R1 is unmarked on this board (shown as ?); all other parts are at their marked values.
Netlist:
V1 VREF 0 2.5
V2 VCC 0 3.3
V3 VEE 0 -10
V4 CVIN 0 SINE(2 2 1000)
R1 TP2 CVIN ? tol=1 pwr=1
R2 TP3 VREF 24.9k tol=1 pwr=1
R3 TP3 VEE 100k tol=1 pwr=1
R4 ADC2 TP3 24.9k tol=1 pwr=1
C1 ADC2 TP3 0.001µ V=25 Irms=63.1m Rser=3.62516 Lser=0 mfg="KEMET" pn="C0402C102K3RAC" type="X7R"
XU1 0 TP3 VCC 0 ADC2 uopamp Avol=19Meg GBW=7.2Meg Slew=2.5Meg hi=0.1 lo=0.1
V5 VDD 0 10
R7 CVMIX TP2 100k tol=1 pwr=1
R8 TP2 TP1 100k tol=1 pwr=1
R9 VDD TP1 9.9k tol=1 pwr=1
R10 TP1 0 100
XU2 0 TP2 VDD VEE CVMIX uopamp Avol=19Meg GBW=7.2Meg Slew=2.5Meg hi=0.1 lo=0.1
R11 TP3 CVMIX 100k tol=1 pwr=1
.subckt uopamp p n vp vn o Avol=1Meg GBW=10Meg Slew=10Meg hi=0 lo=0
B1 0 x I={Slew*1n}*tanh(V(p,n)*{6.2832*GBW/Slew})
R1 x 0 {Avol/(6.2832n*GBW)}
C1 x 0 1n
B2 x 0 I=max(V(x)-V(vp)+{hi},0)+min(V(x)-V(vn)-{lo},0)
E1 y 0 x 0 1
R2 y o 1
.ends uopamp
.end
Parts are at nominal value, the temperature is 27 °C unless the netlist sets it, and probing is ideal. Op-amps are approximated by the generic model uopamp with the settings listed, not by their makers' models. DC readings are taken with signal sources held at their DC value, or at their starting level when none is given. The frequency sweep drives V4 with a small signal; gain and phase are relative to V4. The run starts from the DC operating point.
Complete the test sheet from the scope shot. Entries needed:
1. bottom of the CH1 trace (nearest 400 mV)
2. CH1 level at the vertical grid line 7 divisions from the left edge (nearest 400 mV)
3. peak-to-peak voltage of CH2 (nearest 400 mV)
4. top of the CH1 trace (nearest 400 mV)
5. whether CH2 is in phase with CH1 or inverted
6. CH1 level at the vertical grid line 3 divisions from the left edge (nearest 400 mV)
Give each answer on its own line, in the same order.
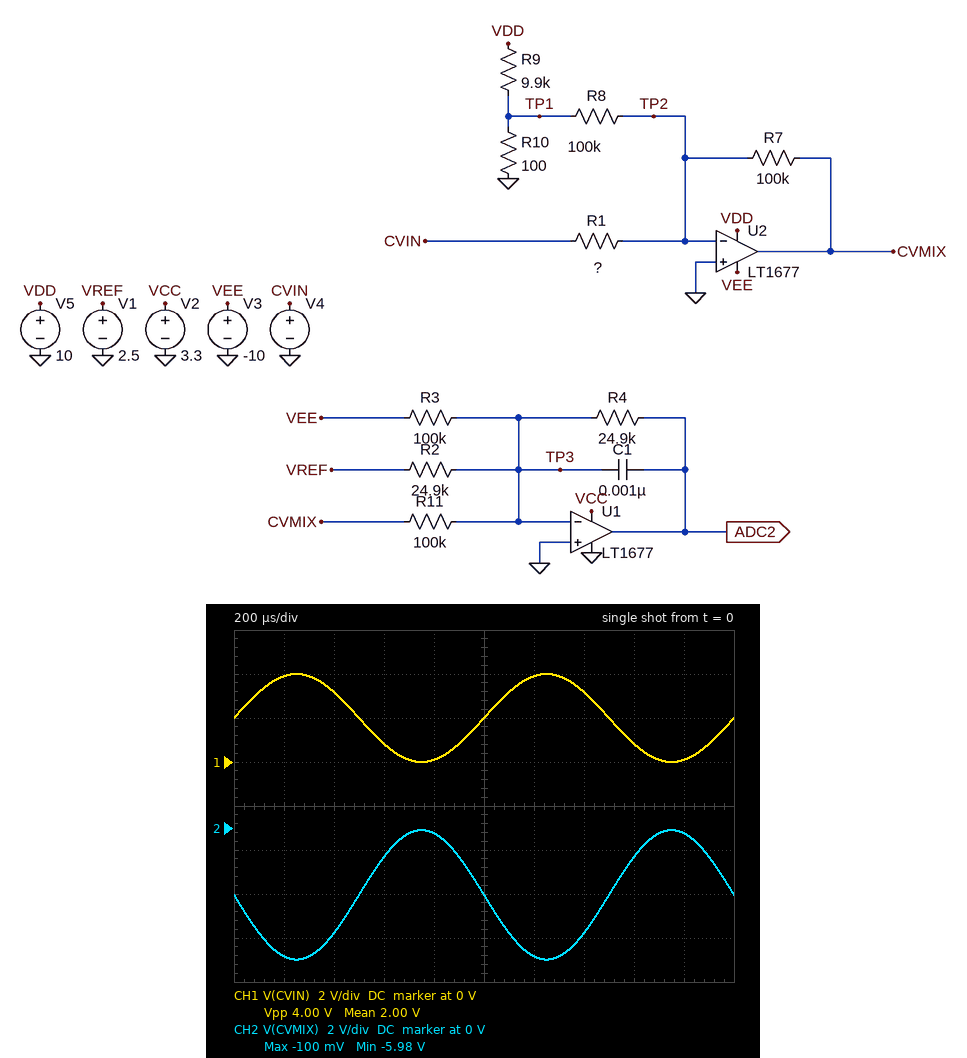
0 V
3.2 V
6.0 V
4.0 V
inverted
800 mV
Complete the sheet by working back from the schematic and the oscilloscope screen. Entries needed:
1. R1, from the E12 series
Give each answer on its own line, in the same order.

68 kΩ
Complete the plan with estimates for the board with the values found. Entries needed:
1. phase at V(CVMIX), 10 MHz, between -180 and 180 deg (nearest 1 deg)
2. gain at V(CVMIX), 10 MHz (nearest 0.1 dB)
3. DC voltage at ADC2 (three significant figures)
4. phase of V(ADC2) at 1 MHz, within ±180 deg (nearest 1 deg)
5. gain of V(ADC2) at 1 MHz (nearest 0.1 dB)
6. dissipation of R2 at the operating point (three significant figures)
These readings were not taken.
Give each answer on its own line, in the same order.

102 deg
-10.5 dB
747 mV
-122 deg
-53.6 dB
251 µW
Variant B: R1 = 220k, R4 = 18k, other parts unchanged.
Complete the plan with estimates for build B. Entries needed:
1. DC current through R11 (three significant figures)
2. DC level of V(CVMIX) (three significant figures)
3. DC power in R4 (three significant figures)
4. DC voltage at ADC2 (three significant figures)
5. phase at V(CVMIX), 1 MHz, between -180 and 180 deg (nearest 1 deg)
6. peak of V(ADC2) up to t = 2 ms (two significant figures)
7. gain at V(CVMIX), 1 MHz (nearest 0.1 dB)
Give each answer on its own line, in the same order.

10.1 µA
-1.01 V
1.69 µW
174 mV
161 deg
340 mV
-7.3 dB
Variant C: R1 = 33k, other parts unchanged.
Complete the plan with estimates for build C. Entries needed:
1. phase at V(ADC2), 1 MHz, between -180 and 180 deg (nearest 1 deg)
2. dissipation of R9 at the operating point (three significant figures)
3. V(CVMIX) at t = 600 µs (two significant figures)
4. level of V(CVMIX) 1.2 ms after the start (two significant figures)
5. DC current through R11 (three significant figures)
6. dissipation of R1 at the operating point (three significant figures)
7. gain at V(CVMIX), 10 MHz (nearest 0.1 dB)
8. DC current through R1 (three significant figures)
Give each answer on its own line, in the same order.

-131 deg
9.90 mW
-2.6 V
-9.9 V
61.6 µA
121 µW
-7.3 dB
60.6 µA
